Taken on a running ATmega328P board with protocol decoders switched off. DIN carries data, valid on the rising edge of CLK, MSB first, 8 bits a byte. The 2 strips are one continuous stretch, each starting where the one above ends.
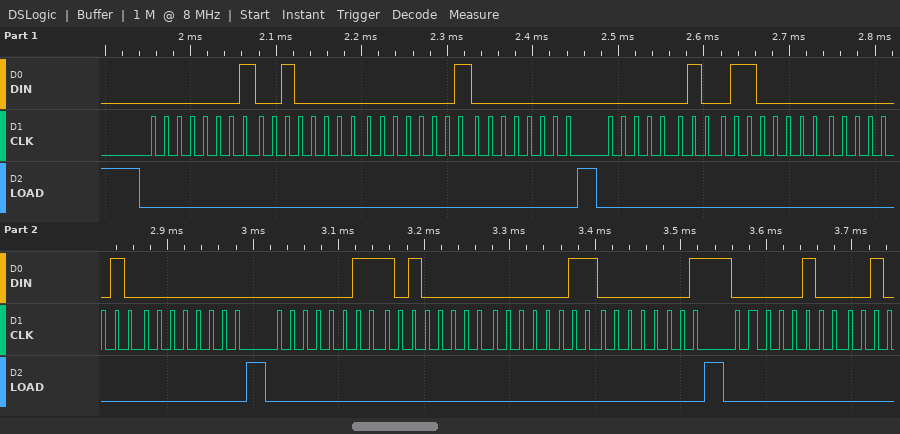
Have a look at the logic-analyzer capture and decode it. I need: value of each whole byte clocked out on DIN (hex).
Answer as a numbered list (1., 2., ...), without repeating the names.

1. 01 20 01 00 02 60 02 00 03 A0 03 01 04
